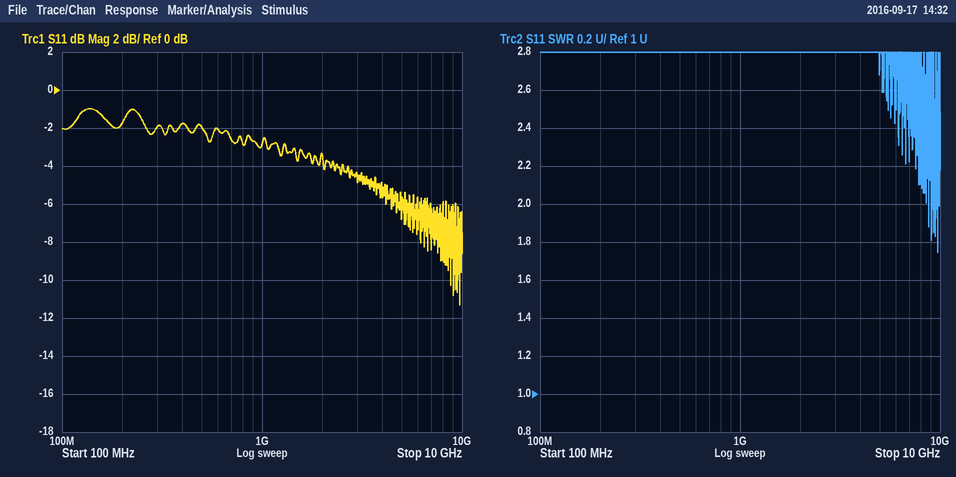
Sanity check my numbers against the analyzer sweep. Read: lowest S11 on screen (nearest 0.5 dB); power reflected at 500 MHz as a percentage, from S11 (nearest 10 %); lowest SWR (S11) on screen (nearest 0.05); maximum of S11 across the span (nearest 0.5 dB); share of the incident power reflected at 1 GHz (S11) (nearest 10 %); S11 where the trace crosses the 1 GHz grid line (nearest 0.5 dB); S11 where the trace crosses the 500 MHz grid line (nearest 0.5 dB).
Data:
-11.5 dB
60 %
1.75
-1.0 dB
50 %
-3.0 dB
-2.0 dB
